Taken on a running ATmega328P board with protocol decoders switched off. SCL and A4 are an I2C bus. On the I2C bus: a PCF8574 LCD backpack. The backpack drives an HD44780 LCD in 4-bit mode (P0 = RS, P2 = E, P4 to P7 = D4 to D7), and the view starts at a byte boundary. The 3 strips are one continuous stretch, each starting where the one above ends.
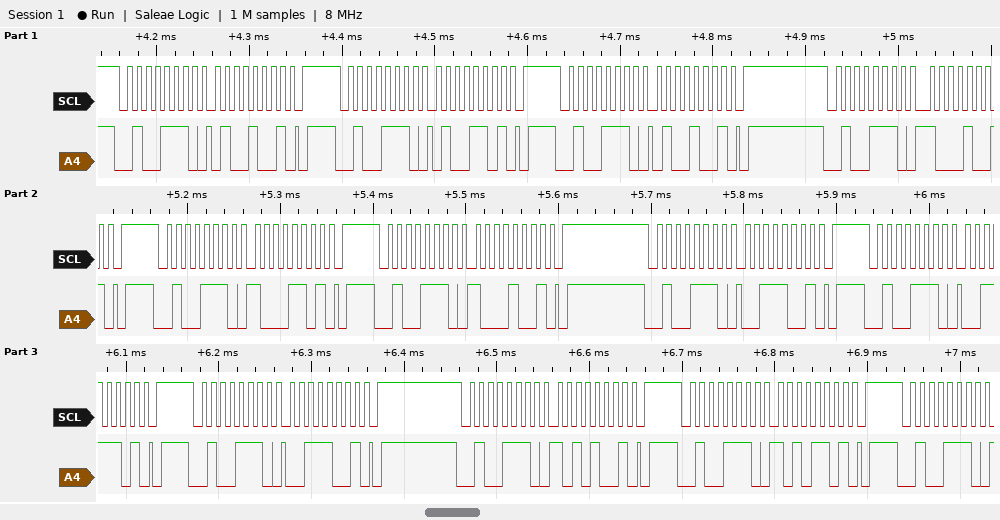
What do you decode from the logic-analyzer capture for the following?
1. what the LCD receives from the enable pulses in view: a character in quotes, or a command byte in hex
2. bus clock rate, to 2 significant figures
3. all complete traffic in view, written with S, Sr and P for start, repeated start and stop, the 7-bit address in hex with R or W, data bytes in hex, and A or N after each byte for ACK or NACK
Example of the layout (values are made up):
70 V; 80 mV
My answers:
'H'; 100 kHz; S 27W A 49 A P S 27W A 4D A P S 27W A 49 A P S 27W A 89 A P S 27W A 8D A P S 27W A 89 A P S 27W A 39 A P S 27W A 3D A P S 27W A 39 A P S 27W A A9 A P S 27W A AD A P S 27W A
